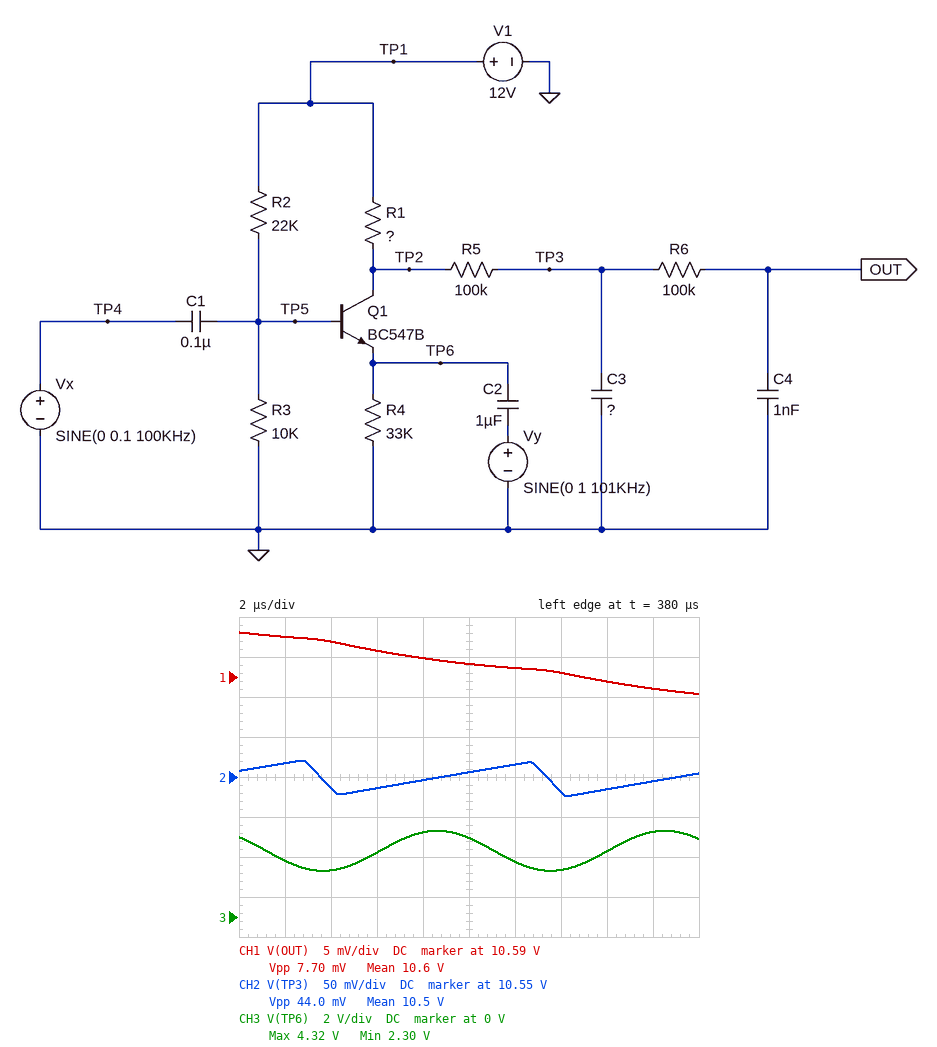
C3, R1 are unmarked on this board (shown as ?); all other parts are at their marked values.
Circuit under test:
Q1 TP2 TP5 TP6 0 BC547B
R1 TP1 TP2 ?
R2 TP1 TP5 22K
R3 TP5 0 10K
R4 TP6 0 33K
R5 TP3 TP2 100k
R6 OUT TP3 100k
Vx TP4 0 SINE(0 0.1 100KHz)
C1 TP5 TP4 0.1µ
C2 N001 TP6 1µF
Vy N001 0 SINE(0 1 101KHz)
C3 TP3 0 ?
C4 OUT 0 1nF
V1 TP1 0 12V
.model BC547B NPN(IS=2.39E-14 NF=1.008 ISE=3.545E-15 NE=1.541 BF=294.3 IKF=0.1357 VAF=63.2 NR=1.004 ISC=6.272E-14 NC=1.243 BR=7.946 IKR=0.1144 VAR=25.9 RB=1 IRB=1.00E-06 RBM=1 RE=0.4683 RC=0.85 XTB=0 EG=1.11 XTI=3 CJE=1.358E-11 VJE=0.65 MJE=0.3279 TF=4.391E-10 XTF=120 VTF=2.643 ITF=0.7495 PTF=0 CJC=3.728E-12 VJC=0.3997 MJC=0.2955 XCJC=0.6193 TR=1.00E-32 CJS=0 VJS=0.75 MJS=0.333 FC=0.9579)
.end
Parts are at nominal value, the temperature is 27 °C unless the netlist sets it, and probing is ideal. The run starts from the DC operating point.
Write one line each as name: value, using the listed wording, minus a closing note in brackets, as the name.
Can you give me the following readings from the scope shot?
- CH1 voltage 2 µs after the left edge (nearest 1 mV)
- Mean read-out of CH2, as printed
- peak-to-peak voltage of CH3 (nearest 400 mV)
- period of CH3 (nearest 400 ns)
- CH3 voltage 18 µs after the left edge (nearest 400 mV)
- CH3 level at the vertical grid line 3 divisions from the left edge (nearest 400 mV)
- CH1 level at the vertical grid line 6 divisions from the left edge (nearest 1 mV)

CH1 voltage 2 µs after the left edge: 10.590 V
Mean read-out of CH2, as printed: 10.5 V
peak-to-peak voltage of CH3: 2.0 V
period of CH3: 10.0 µs
CH3 voltage 18 µs after the left edge: 4.4 V
CH3 level at the vertical grid line 3 divisions from the left edge: 3.2 V
CH1 level at the vertical grid line 6 divisions from the left edge: 10.586 V
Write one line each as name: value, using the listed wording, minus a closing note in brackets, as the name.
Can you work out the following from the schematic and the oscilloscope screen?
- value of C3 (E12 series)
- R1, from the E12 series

value of C3: 2.7 nF
R1, from the E12 series: 12 kΩ
